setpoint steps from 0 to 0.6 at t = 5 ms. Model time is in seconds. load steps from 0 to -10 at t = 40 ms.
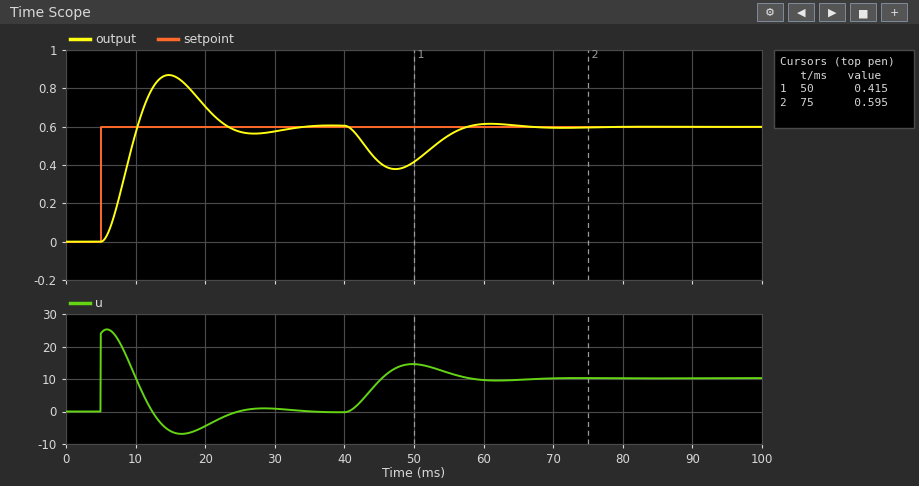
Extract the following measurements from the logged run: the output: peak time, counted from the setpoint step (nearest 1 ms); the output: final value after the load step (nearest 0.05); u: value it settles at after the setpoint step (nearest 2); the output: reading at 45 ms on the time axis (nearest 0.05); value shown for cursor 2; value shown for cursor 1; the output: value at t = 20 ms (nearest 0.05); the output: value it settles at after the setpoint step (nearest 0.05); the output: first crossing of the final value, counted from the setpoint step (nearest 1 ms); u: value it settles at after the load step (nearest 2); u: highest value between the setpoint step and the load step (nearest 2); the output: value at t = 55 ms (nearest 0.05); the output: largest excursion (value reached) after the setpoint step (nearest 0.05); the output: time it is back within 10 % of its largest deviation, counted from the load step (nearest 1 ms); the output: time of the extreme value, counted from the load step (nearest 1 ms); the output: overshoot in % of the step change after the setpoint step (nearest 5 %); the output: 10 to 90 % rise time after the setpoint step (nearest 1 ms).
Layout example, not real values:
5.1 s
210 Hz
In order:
10 ms
0.60
0
0.40
0.595
0.415
0.70
0.60
5 ms
10
26
0.55
0.85
16 ms
7 ms
45 %
4 ms
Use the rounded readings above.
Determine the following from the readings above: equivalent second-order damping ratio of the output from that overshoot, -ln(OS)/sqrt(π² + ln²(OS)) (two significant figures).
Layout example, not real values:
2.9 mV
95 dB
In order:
0.25
